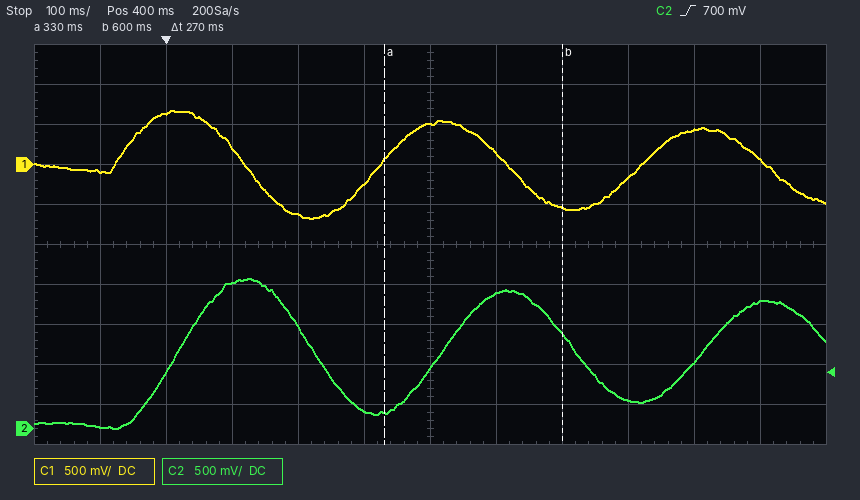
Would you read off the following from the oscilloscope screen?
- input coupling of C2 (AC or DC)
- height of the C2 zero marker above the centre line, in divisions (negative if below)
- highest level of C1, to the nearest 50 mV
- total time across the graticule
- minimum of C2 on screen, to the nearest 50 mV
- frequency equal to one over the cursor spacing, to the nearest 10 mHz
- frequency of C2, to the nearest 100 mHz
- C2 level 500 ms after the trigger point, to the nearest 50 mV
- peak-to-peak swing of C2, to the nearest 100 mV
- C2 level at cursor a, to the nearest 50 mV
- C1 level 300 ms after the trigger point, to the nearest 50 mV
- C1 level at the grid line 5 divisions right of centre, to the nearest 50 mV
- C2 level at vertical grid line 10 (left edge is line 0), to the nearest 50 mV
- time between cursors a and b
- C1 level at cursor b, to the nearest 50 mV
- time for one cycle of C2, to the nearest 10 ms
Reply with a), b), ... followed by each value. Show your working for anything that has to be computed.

a) DC
b) -4.6 div
c) 700 mV
d) 1.2 s
e) 0 mV
f) 1 / 270 ms ≈ 3.70 Hz
g) 1 / 400 ms ≈ 2.5 Hz
h) 1.70 V
i) 1.90 V
j) 200 mV
k) -250 mV
l) 50 mV
m) 850 mV
n) 270 ms
o) -550 mV
p) 400 ms
